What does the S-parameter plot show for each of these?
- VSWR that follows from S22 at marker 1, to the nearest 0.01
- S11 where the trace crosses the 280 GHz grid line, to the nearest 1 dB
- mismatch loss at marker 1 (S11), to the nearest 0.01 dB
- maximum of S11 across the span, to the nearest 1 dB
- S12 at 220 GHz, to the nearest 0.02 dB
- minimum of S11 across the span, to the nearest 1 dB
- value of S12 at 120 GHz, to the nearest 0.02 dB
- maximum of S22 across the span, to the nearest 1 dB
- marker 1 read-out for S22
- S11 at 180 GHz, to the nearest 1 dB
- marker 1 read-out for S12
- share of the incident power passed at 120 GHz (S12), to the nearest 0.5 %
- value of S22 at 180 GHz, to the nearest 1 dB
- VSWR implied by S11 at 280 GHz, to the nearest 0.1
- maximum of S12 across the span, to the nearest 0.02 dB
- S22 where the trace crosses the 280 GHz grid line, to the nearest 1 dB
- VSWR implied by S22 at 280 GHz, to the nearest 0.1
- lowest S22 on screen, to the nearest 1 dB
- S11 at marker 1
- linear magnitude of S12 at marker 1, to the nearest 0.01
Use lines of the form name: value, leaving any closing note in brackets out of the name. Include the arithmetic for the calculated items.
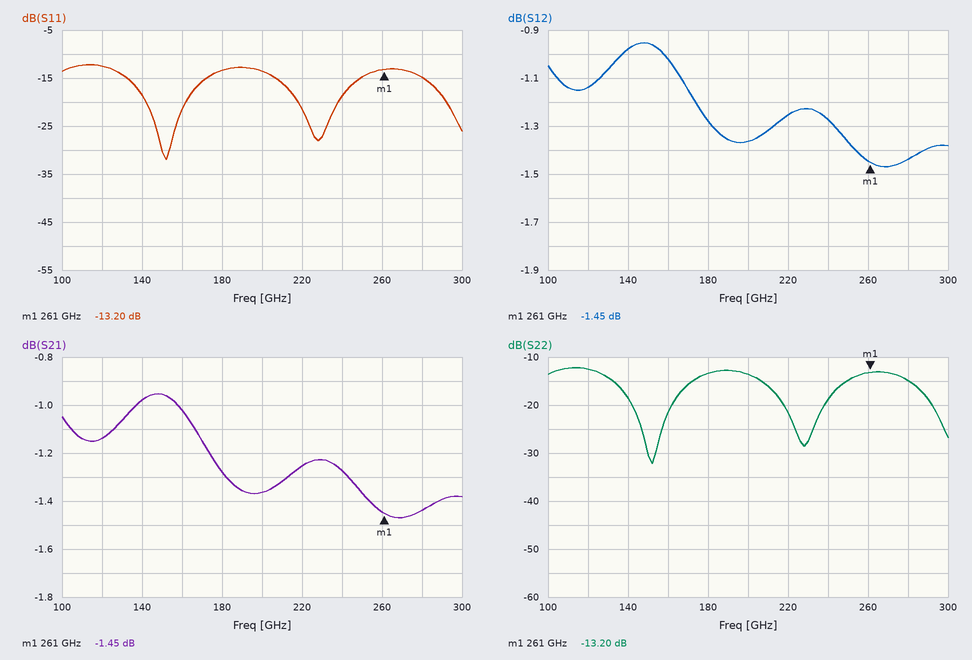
VSWR that follows from S22 at marker 1, to the nearest 0.01: (1 + 0.2188)/(1 − 0.2188) ≈ 1.56
S11 where the trace crosses the 280 GHz grid line, to the nearest 1 dB: -15 dB
mismatch loss at marker 1 (S11), to the nearest 0.01 dB: −10 log10(1 − 10^(-13.2/10)) ≈ 0.21 dB
maximum of S11 across the span, to the nearest 1 dB: -12 dB
S12 at 220 GHz, to the nearest 0.02 dB: -1.26 dB
minimum of S11 across the span, to the nearest 1 dB: -32 dB
value of S12 at 120 GHz, to the nearest 0.02 dB: -1.14 dB
maximum of S22 across the span, to the nearest 1 dB: -12 dB
marker 1 read-out for S22: -13.20 dB
S11 at 180 GHz, to the nearest 1 dB: -13 dB
marker 1 read-out for S12: -1.45 dB
share of the incident power passed at 120 GHz (S12), to the nearest 0.5 %: 10^(-1.14/10) ≈ 76.9 %, so 77.0 % to the nearest 0.5 %
value of S22 at 180 GHz, to the nearest 1 dB: -13 dB
VSWR implied by S11 at 280 GHz, to the nearest 0.1: |Γ| = 10^(-15/20) = 0.1778; VSWR = (1 + 0.1778)/(1 − 0.1778) ≈ 1.4
maximum of S12 across the span, to the nearest 0.02 dB: -0.96 dB
S22 where the trace crosses the 280 GHz grid line, to the nearest 1 dB: -15 dB
VSWR implied by S22 at 280 GHz, to the nearest 0.1: |Γ| = 10^(-15/20) = 0.1778; VSWR = (1 + 0.1778)/(1 − 0.1778) ≈ 1.4
lowest S22 on screen, to the nearest 1 dB: -32 dB
S11 at marker 1: -13.20 dB
linear magnitude of S12 at marker 1, to the nearest 0.01: 10^(-1.45/20) ≈ 0.85
